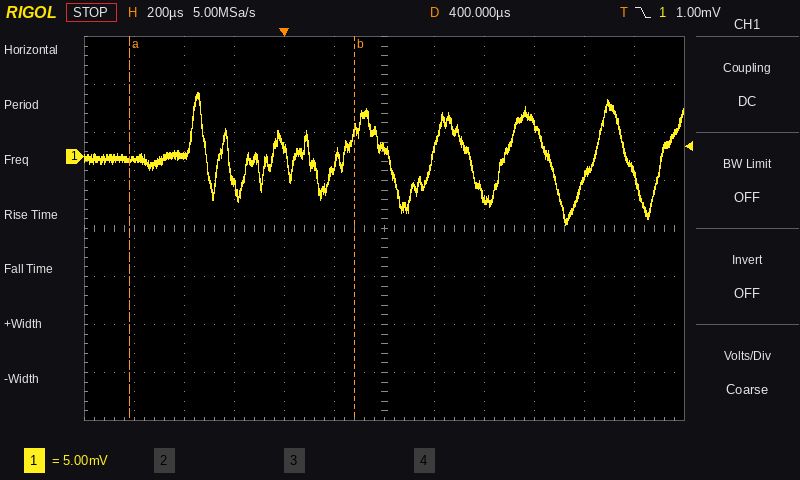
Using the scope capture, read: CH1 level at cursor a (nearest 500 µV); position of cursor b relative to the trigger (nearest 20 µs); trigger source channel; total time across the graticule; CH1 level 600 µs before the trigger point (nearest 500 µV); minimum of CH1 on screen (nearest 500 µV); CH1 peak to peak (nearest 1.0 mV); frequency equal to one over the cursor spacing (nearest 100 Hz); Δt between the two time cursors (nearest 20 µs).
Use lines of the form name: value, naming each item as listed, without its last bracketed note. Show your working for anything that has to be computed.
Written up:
CH1 level at cursor a: -500 µV
position of cursor b relative to the trigger: +280 µs
trigger source channel: CH1
total time across the graticule: 2.4 ms
CH1 level 600 µs before the trigger point: -500 µV
minimum of CH1 on screen: -7.0 mV
CH1 peak to peak: 14.0 mV
frequency equal to one over the cursor spacing: 1 / 900 µs ≈ 1.1 kHz
Δt between the two time cursors: 900 µs
